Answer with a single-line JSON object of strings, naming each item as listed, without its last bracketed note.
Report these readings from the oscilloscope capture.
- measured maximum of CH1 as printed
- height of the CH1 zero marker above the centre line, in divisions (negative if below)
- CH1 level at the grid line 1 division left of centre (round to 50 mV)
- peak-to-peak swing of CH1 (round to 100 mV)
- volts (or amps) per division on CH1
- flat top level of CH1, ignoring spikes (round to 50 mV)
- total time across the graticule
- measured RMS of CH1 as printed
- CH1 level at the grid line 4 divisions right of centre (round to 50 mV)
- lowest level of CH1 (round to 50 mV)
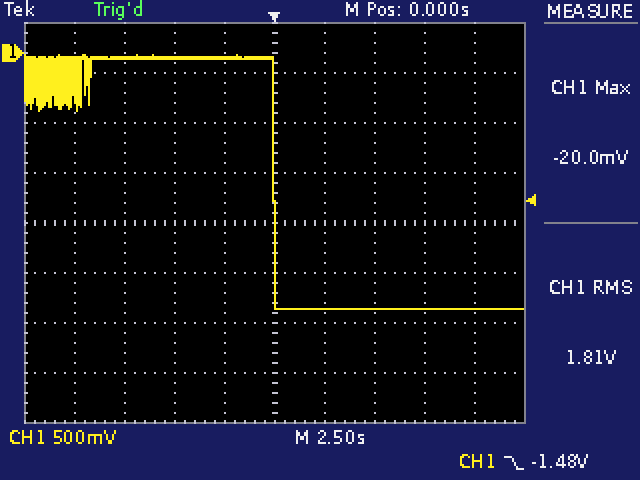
{"measured maximum of CH1 as printed": "-20.0 mV", "height of the CH1 zero marker above the centre line, in divisions": "+3.4 div", "CH1 level at the grid line 1 division left of centre": "-50 mV", "peak-to-peak swing of CH1": "2.50 V", "volts (or amps) per division on CH1": "500 mV", "flat top level of CH1, ignoring spikes": "-50 mV", "total time across the graticule": "25 s", "measured RMS of CH1 as printed": "1.81 V", "CH1 level at the grid line 4 divisions right of centre": "-2.55 V", "lowest level of CH1": "-2.55 V"}
